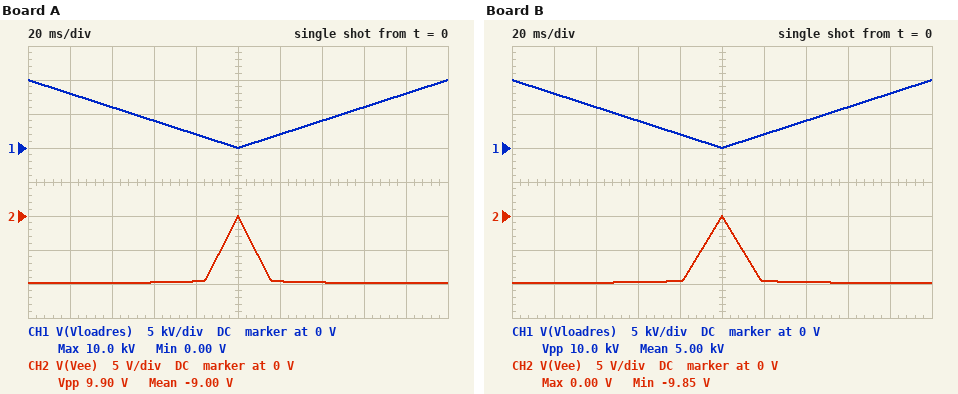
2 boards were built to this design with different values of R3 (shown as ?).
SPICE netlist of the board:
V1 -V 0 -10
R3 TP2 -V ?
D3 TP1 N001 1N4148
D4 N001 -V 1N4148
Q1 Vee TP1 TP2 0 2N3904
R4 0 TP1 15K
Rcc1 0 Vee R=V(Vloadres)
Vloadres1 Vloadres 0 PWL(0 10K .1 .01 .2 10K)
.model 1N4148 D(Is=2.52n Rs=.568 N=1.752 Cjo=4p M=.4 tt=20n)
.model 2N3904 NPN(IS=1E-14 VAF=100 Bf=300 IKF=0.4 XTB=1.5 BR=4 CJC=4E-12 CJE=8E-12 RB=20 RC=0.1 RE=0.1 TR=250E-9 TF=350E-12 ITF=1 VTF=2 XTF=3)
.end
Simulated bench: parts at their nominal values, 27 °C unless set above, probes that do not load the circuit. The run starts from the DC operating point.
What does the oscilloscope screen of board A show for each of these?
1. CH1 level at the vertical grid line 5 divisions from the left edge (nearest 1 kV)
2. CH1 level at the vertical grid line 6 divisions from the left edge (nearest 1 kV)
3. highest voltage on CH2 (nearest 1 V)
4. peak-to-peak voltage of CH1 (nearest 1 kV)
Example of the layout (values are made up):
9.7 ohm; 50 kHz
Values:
0 V; 2 kV; 0 V; 10 kV
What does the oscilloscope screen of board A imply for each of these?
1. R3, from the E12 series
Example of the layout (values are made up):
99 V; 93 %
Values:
68 Ω
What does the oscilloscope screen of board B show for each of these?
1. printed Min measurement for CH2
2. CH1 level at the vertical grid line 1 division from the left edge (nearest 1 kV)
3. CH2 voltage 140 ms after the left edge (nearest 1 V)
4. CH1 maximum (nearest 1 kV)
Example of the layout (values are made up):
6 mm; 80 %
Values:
-9.85 V; 8 kV; -10 V; 10 kV
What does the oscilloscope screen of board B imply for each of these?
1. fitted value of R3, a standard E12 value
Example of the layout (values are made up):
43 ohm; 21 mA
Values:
82 Ω
